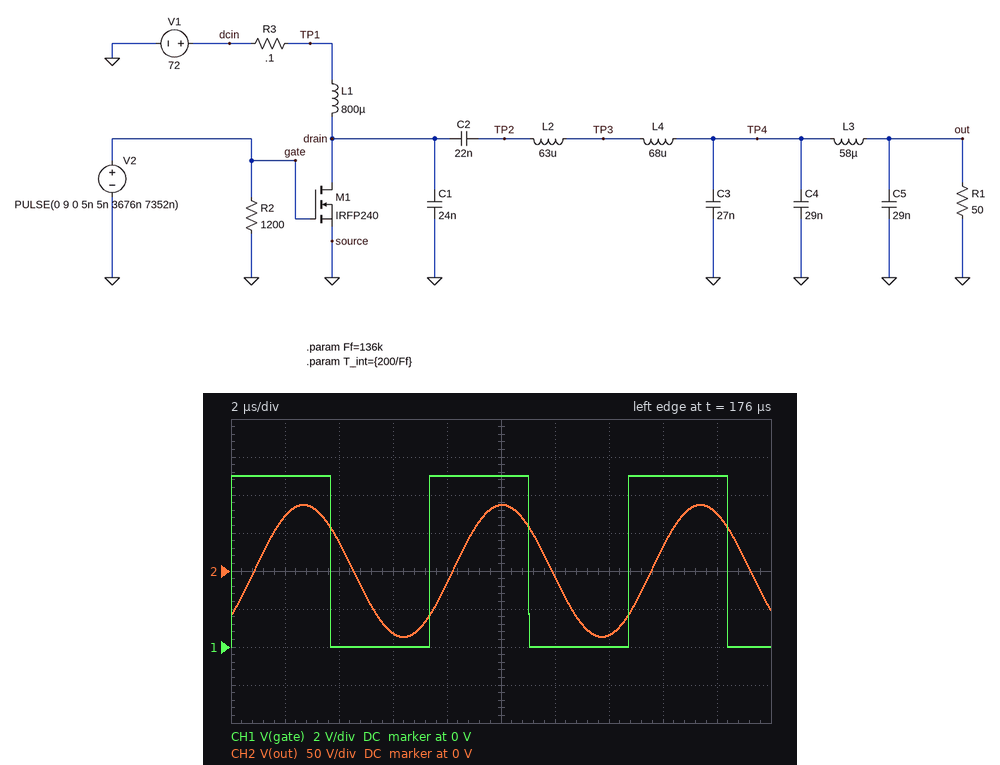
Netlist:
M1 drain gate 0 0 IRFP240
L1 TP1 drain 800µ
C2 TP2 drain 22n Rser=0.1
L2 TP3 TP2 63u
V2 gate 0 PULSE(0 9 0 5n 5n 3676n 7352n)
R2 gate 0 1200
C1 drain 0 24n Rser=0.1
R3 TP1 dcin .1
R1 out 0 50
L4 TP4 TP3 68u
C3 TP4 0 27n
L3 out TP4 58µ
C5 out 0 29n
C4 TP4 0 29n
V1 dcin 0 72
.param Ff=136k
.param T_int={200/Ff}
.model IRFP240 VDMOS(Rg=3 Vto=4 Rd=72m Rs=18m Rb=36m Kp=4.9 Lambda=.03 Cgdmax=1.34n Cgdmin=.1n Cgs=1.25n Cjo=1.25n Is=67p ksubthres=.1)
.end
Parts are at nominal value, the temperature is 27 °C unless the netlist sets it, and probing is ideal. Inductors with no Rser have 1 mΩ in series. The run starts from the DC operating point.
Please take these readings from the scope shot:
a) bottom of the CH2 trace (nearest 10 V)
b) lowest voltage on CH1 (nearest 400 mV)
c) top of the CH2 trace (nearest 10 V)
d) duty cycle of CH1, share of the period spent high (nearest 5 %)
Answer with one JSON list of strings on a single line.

["-90 V", "0 V", "90 V", "50 %"]
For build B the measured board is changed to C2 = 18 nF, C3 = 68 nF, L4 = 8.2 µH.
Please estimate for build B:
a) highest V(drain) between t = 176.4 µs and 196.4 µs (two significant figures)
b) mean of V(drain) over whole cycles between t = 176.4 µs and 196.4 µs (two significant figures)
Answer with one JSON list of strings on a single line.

["410 V", "67 V"]
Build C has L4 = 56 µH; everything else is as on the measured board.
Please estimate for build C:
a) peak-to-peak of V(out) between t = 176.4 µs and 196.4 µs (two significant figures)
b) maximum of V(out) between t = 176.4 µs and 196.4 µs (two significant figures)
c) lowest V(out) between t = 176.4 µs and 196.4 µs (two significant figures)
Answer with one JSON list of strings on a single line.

["220 V", "110 V", "-110 V"]
